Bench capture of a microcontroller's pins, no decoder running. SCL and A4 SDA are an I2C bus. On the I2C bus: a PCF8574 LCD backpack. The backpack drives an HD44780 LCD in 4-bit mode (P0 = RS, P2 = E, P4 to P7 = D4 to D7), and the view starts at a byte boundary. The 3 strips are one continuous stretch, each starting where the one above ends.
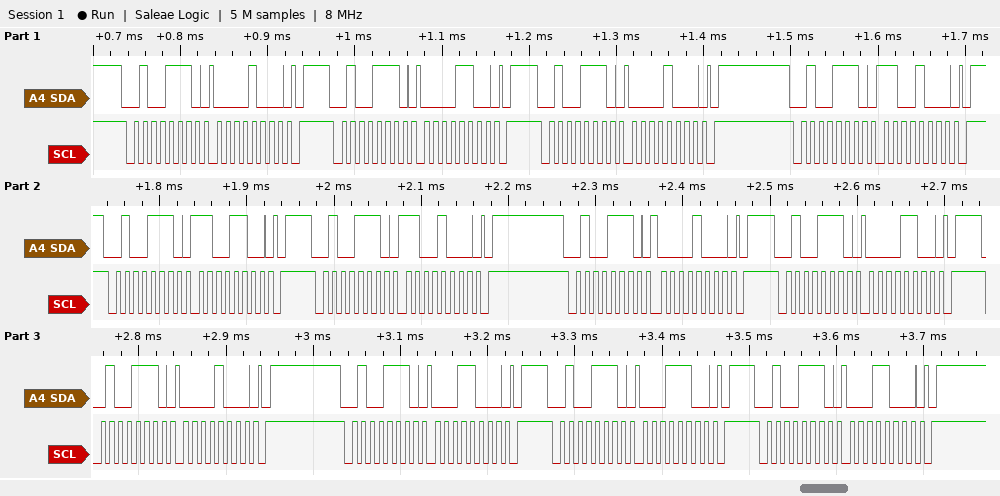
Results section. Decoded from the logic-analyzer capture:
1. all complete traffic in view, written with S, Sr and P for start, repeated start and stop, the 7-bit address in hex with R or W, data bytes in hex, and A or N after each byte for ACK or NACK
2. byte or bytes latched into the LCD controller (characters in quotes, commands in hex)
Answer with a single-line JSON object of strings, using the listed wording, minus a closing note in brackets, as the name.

{"all complete traffic in view, written with S, Sr and P for start, repeated start and stop, the 7-bit address in hex with R or W, data bytes in hex, and A or N after each byte for ACK or NACK": "S 27W A 08 A P S 27W A 0C A P S 27W A 08 A P S 27W A C8 A P S 27W A CC A P S 27W A C8 A P S 27W A 08 A P S 27W A 0C A P S 27W A 08 A P S 27W A 18 A P S 27W A 1C A P S 27W A 18 A P", "byte or bytes latched into the LCD controller": "0x0C 0x01"}
